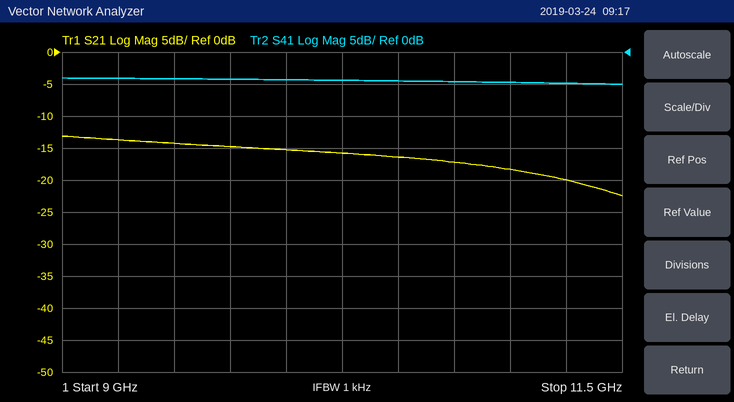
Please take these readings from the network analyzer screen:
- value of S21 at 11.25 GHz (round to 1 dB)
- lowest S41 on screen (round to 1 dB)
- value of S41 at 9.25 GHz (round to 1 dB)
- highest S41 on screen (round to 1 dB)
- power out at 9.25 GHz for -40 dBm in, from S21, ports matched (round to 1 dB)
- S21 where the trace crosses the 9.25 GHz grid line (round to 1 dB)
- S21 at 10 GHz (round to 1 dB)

-20 dB
-5 dB
-4 dB
-4 dB
-54 dBm
-14 dB
-15 dB
